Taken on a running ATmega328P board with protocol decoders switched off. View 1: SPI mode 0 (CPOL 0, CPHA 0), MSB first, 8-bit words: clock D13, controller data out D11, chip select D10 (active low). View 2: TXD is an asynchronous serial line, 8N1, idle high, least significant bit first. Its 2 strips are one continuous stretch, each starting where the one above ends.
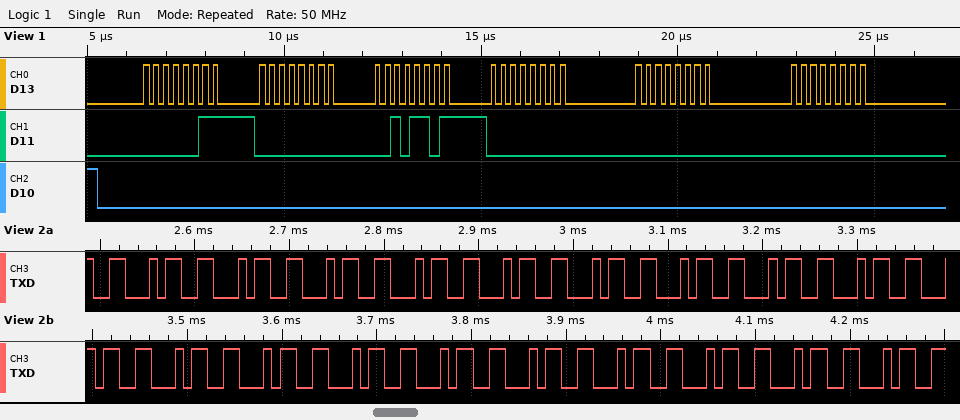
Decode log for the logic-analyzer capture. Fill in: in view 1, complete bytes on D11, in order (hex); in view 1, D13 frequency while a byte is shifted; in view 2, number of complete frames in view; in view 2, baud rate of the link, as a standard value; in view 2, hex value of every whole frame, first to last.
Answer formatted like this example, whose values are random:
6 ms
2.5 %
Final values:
03 00 2D 00 00 00
4 MHz
19
115200 baud
0x46 0x46 0x46 0x46 0x46 0x46 0x46 0x46 0x46 0x46 0x46 0x46 0x46 0x46 0x46 0x46 0x46 0x46 0x46
